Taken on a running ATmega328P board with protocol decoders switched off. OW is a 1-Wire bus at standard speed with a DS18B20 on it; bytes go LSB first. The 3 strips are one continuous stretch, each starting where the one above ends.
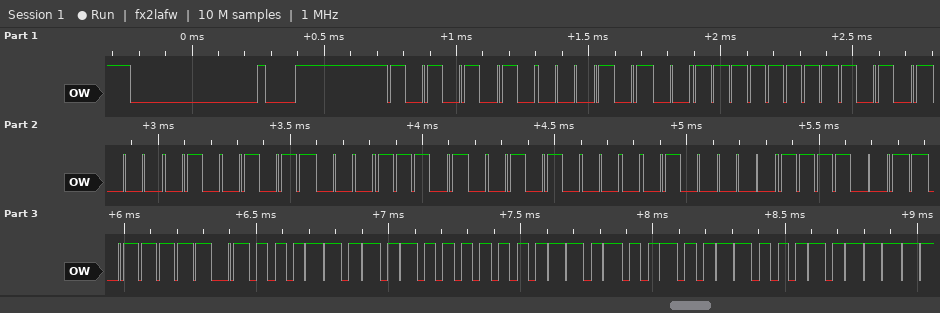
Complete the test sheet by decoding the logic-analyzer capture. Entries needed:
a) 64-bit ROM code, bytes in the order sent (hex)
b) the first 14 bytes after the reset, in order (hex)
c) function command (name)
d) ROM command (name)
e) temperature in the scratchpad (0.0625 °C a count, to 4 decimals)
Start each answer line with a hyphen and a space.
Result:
- 28 FF 15 D2 B8 14 04 CF
- 55 28 FF 15 D2 B8 14 04 CF BE 58 01 4B 46
- Read Scratchpad
- Match ROM
- 21.5000 °C
